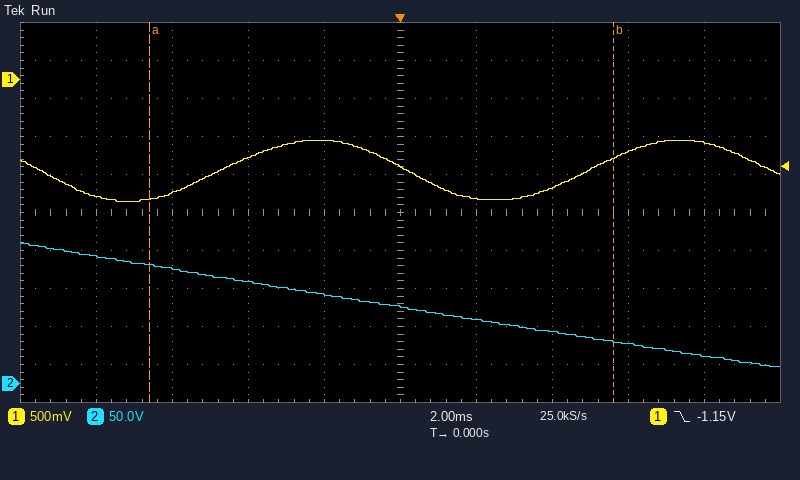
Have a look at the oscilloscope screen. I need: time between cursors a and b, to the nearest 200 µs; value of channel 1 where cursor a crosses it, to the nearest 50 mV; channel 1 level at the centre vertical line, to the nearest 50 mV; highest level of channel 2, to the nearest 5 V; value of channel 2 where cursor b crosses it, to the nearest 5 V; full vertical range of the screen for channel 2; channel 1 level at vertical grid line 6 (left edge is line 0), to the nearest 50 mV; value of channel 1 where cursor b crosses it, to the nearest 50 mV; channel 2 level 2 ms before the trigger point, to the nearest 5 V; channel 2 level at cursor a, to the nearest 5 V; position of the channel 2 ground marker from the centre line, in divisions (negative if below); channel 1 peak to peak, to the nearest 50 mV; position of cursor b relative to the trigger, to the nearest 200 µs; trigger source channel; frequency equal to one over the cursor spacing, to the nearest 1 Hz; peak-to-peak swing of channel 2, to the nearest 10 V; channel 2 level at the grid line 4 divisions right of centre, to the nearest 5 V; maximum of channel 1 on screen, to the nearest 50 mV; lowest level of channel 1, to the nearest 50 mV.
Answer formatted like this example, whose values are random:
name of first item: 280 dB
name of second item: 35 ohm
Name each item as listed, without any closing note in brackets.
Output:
time between cursors a and b, to the nearest 200 µs: 12.2 ms
value of channel 1 where cursor a crosses it, to the nearest 50 mV: -1.55 V
channel 1 level at the centre vertical line, to the nearest 50 mV: -1.15 V
highest level of channel 2, to the nearest 5 V: 185 V
value of channel 2 where cursor b crosses it, to the nearest 5 V: 55 V
full vertical range of the screen for channel 2: 500 V
channel 1 level at vertical grid line 6 (left edge is line 0), to the nearest 50 mV: -1.55 V
value of channel 1 where cursor b crosses it, to the nearest 50 mV: -1.05 V
channel 2 level 2 ms before the trigger point, to the nearest 5 V: 115 V
channel 2 level at cursor a, to the nearest 5 V: 155 V
position of the channel 2 ground marker from the centre line, in divisions: -4.5 div
channel 1 peak to peak, to the nearest 50 mV: 800 mV
position of cursor b relative to the trigger, to the nearest 200 µs: +5.6 ms
trigger source channel: channel 1
frequency equal to one over the cursor spacing, to the nearest 1 Hz: 82 Hz
peak-to-peak swing of channel 2, to the nearest 10 V: 160 V
channel 2 level at the grid line 4 divisions right of centre, to the nearest 5 V: 35 V
maximum of channel 1 on screen, to the nearest 50 mV: -800 mV
lowest level of channel 1, to the nearest 50 mV: -1.60 V
